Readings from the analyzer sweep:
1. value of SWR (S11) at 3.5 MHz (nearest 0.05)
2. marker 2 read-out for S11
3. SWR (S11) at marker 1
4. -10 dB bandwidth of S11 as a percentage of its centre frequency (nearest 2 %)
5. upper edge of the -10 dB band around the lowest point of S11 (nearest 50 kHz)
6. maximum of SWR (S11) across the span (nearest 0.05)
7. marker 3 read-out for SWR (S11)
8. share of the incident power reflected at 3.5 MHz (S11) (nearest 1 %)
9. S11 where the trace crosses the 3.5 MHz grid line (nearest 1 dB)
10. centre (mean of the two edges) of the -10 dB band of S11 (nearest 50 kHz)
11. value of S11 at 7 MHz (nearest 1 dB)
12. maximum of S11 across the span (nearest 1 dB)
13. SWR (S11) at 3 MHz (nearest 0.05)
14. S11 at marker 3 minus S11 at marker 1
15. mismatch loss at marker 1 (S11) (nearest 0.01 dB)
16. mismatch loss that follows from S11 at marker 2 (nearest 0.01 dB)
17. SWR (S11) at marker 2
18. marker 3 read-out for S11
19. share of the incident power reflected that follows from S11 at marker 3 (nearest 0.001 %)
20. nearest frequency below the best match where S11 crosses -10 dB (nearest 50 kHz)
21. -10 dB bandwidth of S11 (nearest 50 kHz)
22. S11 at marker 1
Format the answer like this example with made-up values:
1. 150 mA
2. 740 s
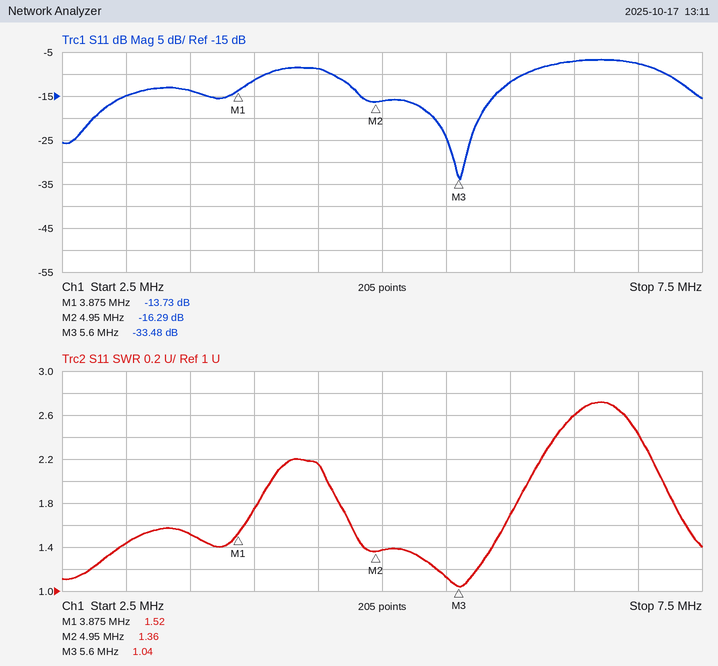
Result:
1. 1.50
2. -16.29 dB
3. 1.52
4. 28 %
5. 6.10 MHz
6. 2.70
7. 1.04
8. 4 %
9. -14 dB
10. 5.35 MHz
11. -8 dB
12. -7 dB
13. 1.45
14. -19.75 dB
15. 0.19 dB
16. 0.10 dB
17. 1.36
18. -33.48 dB
19. 0.045 %
20. 4.60 MHz
21. 1.50 MHz
22. -13.73 dB
